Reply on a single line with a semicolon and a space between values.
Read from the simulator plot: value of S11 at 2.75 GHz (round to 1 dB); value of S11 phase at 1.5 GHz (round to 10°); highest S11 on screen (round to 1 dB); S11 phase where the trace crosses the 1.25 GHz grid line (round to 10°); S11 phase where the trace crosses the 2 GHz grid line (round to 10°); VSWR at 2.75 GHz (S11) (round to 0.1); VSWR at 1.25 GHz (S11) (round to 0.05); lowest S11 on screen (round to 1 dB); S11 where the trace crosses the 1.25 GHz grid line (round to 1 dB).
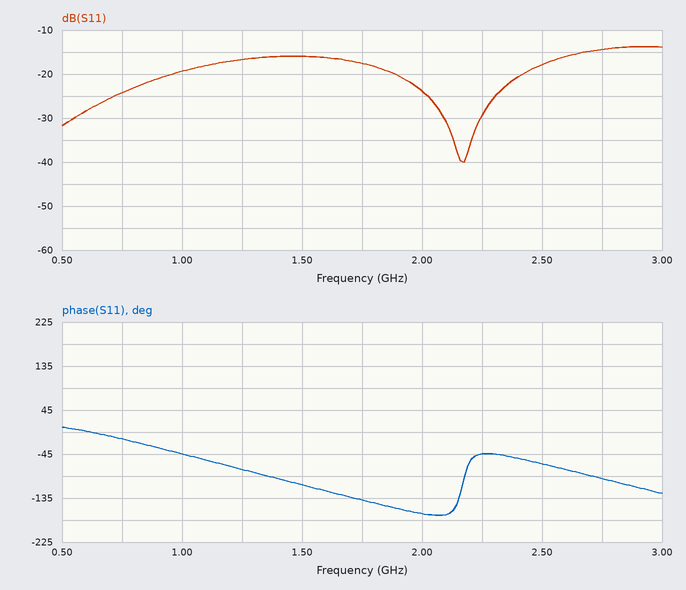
-14 dB; -110°; -14 dB; -80°; -170°; 1.5; 1.35; -40 dB; -17 dB
